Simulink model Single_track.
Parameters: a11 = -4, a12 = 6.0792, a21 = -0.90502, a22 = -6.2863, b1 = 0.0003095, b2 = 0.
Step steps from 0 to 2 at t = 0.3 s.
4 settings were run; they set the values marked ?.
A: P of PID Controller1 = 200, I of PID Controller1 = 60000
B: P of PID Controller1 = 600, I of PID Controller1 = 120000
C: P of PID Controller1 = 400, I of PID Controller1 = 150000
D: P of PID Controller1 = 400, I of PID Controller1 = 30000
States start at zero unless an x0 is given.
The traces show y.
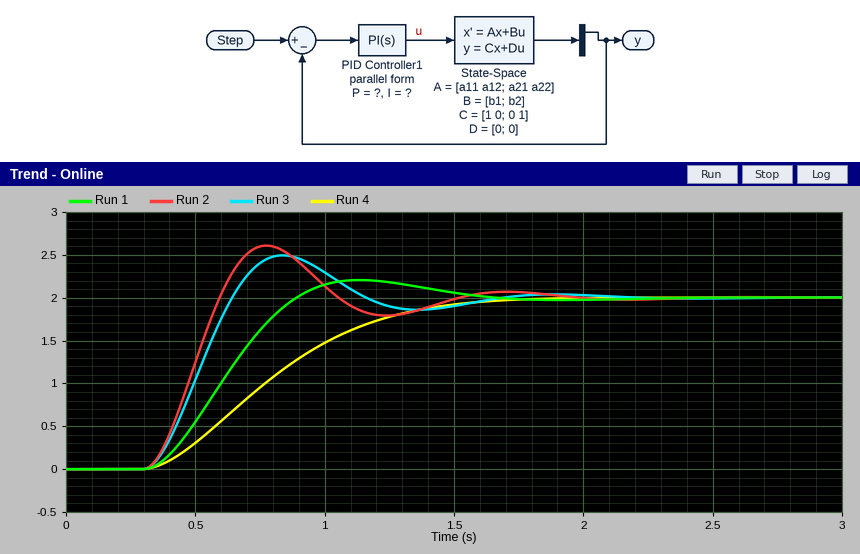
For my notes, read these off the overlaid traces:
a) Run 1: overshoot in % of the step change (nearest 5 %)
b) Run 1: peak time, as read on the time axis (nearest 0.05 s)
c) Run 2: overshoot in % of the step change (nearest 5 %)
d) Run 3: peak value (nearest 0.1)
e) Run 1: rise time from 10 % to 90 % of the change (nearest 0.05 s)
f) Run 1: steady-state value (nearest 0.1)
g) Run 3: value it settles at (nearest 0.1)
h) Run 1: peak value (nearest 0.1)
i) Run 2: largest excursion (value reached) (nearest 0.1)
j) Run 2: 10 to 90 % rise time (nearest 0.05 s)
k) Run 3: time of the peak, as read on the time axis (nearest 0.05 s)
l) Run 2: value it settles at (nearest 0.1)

10 %
1.15 s
30 %
2.5
0.40 s
2.0
2.0
2.2
2.6
0.20 s
0.85 s
2.0
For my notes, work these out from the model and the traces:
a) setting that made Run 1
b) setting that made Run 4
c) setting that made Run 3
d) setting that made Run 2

A
D
B
C
